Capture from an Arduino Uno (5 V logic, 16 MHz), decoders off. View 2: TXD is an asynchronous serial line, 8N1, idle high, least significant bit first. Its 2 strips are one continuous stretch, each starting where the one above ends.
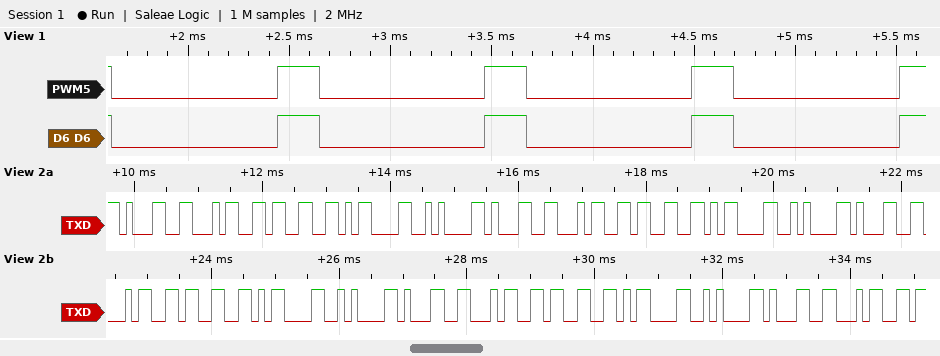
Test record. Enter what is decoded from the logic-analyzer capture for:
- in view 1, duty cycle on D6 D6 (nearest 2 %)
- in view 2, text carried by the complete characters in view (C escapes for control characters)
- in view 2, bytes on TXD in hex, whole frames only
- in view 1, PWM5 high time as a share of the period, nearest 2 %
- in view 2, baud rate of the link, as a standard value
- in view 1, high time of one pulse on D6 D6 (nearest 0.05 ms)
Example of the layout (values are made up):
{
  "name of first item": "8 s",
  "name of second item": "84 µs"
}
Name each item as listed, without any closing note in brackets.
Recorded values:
{
  "in view 1, duty cycle on D6 D6": "20 %",
  "in view 2, text carried by the complete characters in view": "\"143\\r\\n143\\r\\n143\\r\\n143\\r\\n14\"",
  "in view 2, bytes on TXD in hex, whole frames only": "31 34 33 0D 0A 31 34 33 0D 0A 31 34 33 0D 0A 31 34 33 0D 0A 31 34",
  "in view 1, PWM5 high time as a share of the period, nearest 2 %": "20 %",
  "in view 2, baud rate of the link, as a standard value": "9600 baud",
  "in view 1, high time of one pulse on D6 D6": "0.20 ms"
}
